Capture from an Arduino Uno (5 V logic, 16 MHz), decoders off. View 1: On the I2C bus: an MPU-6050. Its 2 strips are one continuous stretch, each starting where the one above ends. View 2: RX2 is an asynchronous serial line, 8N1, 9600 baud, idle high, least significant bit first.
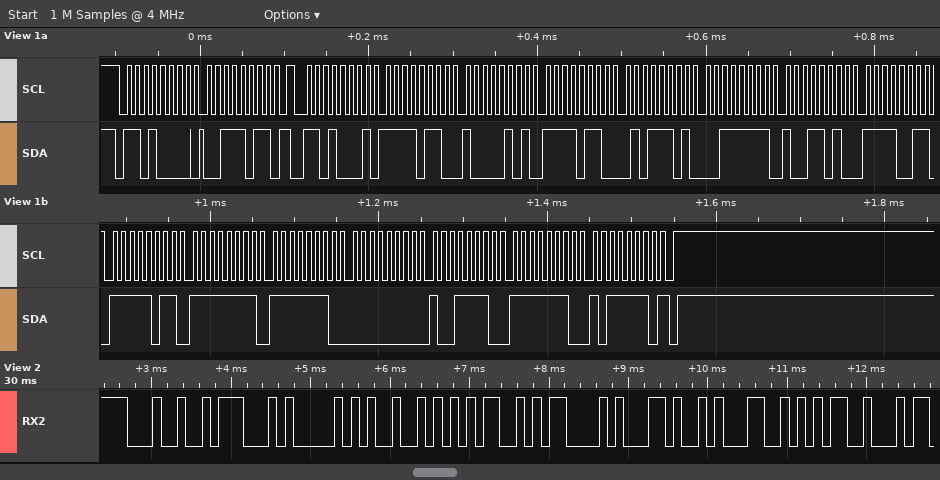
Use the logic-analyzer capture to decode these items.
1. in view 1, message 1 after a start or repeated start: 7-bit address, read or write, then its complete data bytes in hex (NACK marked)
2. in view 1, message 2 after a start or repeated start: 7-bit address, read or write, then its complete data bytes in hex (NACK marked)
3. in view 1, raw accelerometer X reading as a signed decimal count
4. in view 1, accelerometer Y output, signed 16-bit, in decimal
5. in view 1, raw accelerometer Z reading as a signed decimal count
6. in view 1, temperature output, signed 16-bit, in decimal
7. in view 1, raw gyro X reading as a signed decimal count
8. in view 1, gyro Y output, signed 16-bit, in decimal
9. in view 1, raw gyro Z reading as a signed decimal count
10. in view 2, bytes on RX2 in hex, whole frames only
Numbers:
0x68 write: 3B
0x68 read: F6 85 F6 5D 3F 9A F3 FB FF FE 00 9E FE BE NACK
-2427
-2467
16282
-3077
-2
158
-322
24 47 50 52 4D 43 2C 31 35
